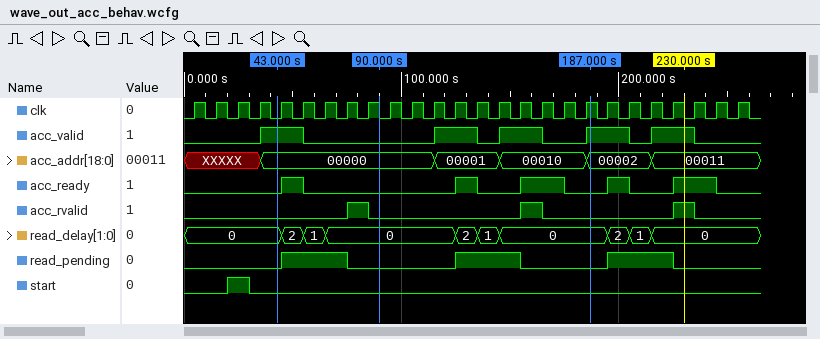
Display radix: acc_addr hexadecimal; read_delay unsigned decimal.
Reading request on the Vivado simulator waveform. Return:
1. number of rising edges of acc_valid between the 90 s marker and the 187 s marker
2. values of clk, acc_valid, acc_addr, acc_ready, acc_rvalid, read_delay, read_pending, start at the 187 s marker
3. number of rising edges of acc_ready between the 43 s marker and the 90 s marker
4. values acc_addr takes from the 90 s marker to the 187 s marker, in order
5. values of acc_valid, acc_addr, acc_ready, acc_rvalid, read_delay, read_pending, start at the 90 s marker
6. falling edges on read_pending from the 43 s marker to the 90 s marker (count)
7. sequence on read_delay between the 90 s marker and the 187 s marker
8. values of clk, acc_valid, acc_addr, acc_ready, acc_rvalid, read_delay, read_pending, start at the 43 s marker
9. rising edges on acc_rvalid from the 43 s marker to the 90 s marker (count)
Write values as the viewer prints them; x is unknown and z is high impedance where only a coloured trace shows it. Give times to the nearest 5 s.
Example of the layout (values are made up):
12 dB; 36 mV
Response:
3; clk=1, acc_valid=1, acc_addr=00002, acc_ready=0, acc_rvalid=0, read_delay=0, read_pending=0, start=0; 1; 00000, 00001, 00010, 00002; acc_valid=0, acc_addr=00000, acc_ready=0, acc_rvalid=0, read_delay=0, read_pending=0, start=0; 1; 0, 2, 1, 0; clk=0, acc_valid=1, acc_addr=00000, acc_ready=0, acc_rvalid=0, read_delay=0, read_pending=0, start=0; 1
